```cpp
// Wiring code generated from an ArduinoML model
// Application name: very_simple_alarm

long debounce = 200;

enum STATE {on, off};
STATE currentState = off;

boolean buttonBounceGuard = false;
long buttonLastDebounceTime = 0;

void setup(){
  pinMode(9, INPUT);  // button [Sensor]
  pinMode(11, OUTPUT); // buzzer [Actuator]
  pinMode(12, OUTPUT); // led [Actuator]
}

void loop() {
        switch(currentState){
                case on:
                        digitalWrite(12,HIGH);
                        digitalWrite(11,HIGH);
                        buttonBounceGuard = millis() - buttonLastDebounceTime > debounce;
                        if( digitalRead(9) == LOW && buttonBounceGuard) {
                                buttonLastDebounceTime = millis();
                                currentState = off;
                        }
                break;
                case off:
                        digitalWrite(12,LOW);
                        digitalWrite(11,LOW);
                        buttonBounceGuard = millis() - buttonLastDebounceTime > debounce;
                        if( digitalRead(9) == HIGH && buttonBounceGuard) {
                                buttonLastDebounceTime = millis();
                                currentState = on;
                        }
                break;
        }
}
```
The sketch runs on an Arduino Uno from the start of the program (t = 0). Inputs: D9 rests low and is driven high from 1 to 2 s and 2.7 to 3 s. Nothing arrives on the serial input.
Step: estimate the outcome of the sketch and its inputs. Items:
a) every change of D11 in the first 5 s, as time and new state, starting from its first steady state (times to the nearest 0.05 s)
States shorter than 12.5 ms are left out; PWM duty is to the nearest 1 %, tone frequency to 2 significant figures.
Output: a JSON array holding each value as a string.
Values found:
["0 s low; 1 s high; 2 s low; 2.7 s high; 3 s low"]
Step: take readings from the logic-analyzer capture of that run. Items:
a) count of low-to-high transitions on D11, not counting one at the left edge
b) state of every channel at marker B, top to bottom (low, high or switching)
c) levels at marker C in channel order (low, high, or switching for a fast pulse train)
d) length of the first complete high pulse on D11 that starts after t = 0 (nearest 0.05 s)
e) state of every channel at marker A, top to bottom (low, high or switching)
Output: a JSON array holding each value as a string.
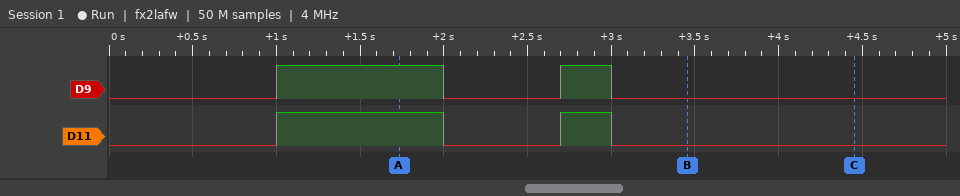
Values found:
["2", "D9 low, D11 low", "D9 low, D11 low", "1.00 s", "D9 high, D11 high"]
